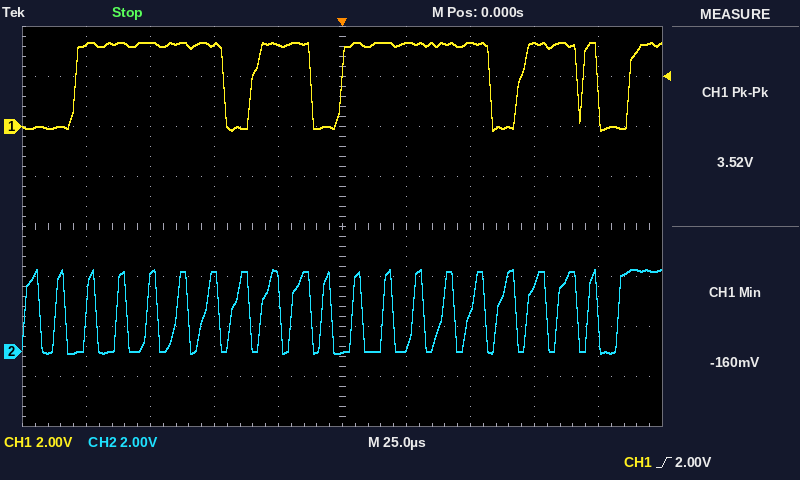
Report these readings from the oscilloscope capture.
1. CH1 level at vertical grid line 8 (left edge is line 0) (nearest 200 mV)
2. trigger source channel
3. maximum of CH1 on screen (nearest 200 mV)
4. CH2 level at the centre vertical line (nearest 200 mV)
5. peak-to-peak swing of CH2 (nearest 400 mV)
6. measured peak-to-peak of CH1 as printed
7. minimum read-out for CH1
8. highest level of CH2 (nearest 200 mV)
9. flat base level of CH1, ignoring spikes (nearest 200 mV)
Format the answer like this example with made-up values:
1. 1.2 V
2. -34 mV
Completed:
1. 3.4 V
2. CH1
3. 3.4 V
4. 0.0 V
5. 3.2 V
6. 3.52 V
7. -160 mV
8. 3.2 V
9. 0.0 V
